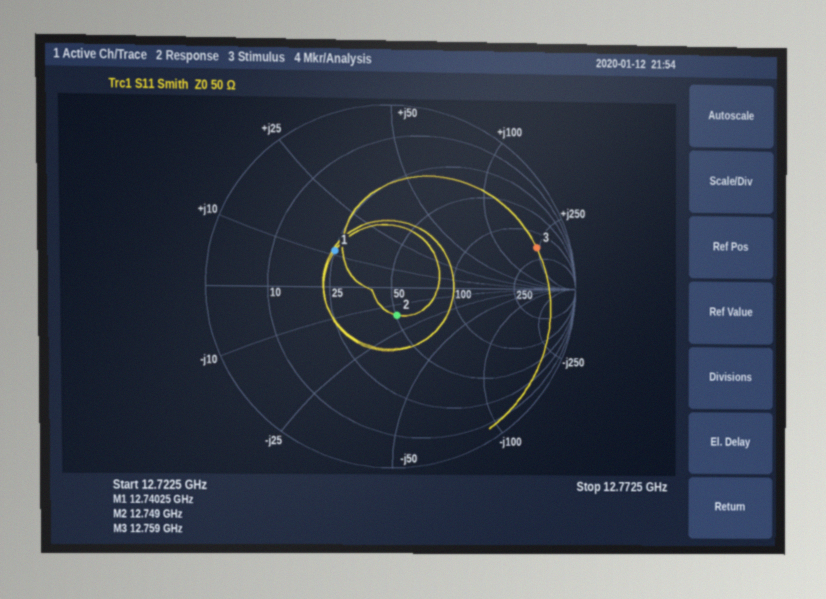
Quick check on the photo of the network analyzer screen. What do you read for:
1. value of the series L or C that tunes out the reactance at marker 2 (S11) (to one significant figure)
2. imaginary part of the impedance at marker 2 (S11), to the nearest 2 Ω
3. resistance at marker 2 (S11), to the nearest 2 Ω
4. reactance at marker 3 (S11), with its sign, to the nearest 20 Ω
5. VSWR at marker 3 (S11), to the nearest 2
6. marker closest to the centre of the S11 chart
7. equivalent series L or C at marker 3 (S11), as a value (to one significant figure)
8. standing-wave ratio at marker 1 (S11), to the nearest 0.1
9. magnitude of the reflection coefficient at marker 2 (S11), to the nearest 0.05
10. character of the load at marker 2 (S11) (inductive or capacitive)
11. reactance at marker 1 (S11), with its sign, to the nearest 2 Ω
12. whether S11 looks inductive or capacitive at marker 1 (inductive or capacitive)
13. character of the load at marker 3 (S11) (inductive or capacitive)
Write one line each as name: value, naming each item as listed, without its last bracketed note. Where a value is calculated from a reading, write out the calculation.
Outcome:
value of the series L or C that tunes out the reactance at marker 2 (S11): L = 16 Ω/(2π × 12.749 GHz) ≈ 200 pH
imaginary part of the impedance at marker 2 (S11), to the nearest 2 Ω: -16 Ω
resistance at marker 2 (S11), to the nearest 2 Ω: 50 Ω
reactance at marker 3 (S11), with its sign, to the nearest 20 Ω: +240 Ω
VSWR at marker 3 (S11), to the nearest 2: 10
marker closest to the centre of the S11 chart: marker 2
equivalent series L or C at marker 3 (S11), as a value: L = 240 Ω/(2π × 12.759 GHz) ≈ 3 nH
standing-wave ratio at marker 1 (S11), to the nearest 0.1: 2.1
magnitude of the reflection coefficient at marker 2 (S11), to the nearest 0.05: 0.15
character of the load at marker 2 (S11): capacitive
reactance at marker 1 (S11), with its sign, to the nearest 2 Ω: +12 Ω
whether S11 looks inductive or capacitive at marker 1: inductive
character of the load at marker 3 (S11): inductive
